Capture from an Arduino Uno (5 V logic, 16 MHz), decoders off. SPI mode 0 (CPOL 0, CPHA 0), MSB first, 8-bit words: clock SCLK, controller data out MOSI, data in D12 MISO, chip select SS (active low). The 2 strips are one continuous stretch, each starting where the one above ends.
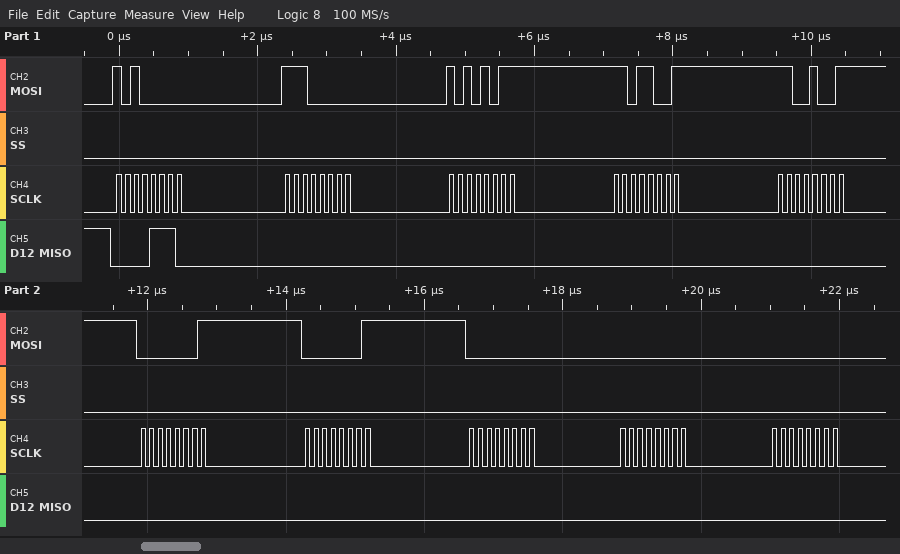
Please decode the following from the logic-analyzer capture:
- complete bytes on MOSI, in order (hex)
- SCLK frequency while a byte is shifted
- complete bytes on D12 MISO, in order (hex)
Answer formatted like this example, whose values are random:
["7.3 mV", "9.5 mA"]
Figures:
["A0 E0 AB D9 C9 01 01 00 00 00", "8 MHz", "0E 00 00 00 00 00 00 00 00 00"]
